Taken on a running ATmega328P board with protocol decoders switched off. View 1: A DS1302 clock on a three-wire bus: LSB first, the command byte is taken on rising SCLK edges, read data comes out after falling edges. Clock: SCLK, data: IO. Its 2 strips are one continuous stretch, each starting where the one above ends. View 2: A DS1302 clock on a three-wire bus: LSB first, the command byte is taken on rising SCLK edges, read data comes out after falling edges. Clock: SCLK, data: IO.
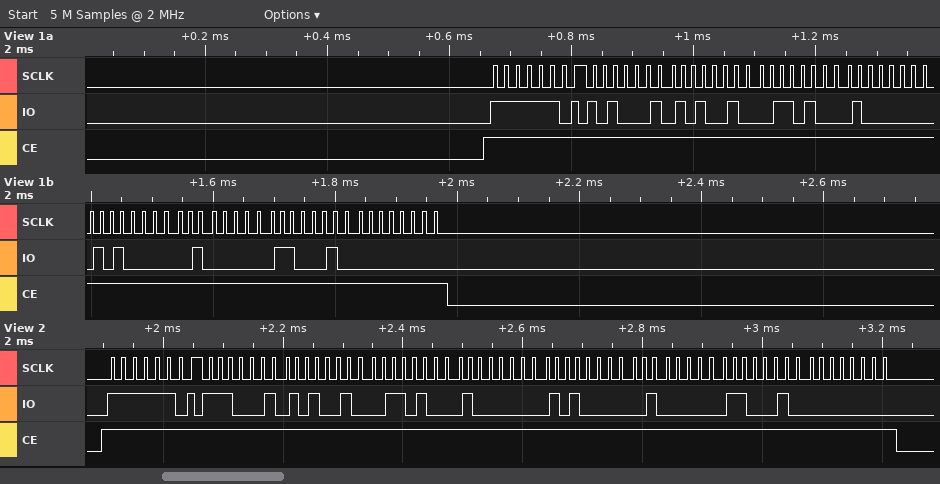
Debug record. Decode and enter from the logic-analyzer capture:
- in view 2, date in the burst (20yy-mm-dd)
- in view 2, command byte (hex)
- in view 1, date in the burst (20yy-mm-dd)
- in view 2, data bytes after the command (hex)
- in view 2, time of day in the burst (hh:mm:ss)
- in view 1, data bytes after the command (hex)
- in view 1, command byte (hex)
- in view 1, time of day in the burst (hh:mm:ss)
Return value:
2023-05-01
0xBF
2023-05-01
47 25 16 01 05 02 23 00
16:25:47
45 25 16 01 05 02 23 00
0xBF
16:25:45
